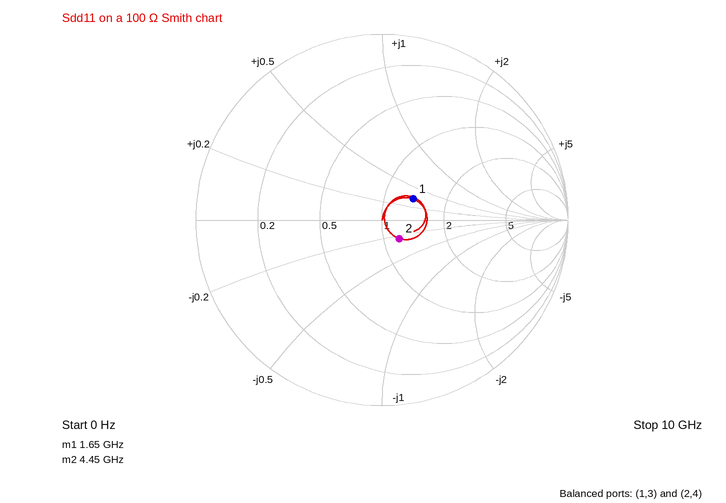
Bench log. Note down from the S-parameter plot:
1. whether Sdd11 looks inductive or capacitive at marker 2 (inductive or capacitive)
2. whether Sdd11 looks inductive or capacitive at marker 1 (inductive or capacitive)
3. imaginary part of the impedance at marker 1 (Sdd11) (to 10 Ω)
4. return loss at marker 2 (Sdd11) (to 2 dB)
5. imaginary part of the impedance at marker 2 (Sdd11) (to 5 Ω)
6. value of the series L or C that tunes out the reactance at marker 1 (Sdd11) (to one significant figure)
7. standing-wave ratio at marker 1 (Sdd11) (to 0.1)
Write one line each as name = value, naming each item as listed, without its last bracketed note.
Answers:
whether Sdd11 looks inductive or capacitive at marker 2 = capacitive
whether Sdd11 looks inductive or capacitive at marker 1 = inductive
imaginary part of the impedance at marker 1 (Sdd11) = +30 Ω
return loss at marker 2 (Sdd11) = 18 dB
imaginary part of the impedance at marker 2 (Sdd11) = -25 Ω
value of the series L or C that tunes out the reactance at marker 1 (Sdd11) = 3 pF
standing-wave ratio at marker 1 (Sdd11) = 1.5
